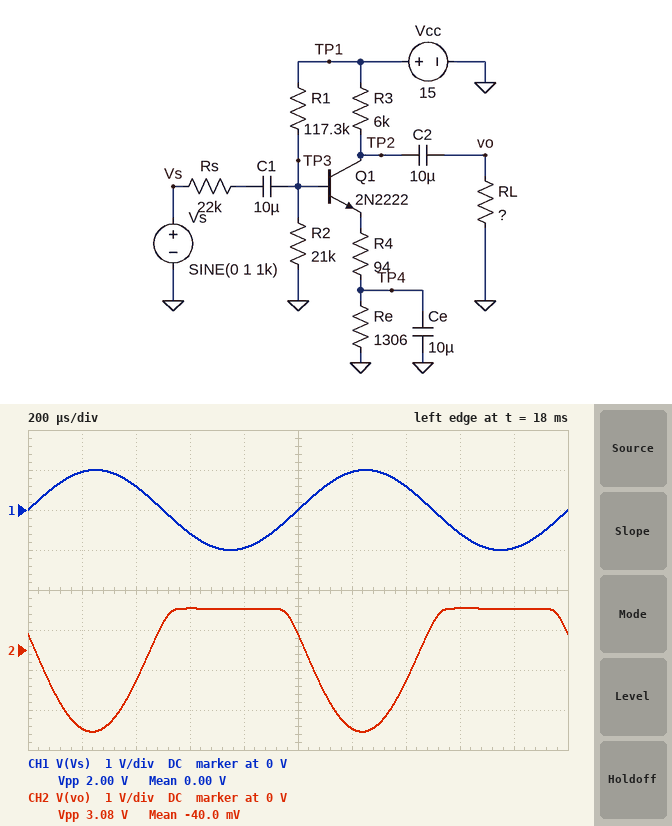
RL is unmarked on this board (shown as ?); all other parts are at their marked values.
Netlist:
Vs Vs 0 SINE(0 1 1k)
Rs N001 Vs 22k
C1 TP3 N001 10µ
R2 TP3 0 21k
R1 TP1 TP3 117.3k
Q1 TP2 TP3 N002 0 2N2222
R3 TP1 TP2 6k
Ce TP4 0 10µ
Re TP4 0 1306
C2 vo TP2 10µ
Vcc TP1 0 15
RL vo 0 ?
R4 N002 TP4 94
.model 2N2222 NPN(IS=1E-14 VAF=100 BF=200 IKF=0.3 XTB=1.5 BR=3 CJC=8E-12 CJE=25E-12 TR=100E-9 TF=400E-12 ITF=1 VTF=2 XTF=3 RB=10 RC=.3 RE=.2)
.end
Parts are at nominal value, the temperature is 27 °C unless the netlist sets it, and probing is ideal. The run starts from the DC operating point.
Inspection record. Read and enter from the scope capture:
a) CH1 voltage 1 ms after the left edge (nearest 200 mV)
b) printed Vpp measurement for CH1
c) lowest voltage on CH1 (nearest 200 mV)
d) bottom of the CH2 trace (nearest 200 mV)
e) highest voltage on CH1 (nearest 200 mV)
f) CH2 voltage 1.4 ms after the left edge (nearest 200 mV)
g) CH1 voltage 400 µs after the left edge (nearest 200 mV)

0 V
2.00 V
-1.0 V
-2.0 V
1.0 V
-800 mV
600 mV
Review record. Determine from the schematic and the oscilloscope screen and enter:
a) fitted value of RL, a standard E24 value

1.1 kΩ
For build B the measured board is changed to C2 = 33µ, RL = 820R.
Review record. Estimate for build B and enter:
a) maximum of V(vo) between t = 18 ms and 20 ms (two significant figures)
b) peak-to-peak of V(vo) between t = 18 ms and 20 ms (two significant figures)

790 mV
2.4 V
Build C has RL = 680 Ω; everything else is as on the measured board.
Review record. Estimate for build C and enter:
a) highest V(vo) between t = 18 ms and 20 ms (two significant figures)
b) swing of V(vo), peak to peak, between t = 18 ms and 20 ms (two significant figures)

680 mV
2.0 V
